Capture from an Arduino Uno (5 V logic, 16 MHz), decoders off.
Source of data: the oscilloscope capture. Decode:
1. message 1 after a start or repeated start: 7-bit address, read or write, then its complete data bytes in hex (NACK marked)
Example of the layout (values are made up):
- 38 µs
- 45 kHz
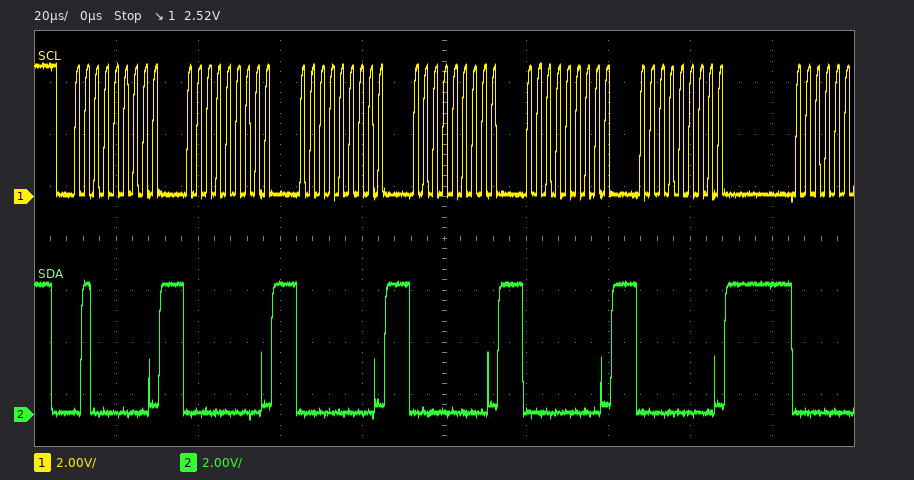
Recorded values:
- 0x20 write: 00 00 00 00 00
